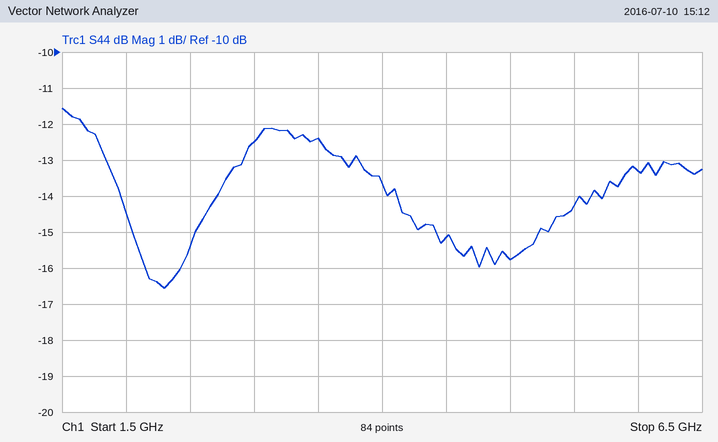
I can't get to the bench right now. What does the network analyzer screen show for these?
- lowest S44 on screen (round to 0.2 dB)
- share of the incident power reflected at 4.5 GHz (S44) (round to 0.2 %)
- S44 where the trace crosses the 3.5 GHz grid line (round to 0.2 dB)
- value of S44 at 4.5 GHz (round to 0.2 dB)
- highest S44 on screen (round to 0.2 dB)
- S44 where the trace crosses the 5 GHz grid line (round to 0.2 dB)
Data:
-16.6 dB
3.0 %
-12.4 dB
-15.2 dB
-11.6 dB
-15.8 dB
